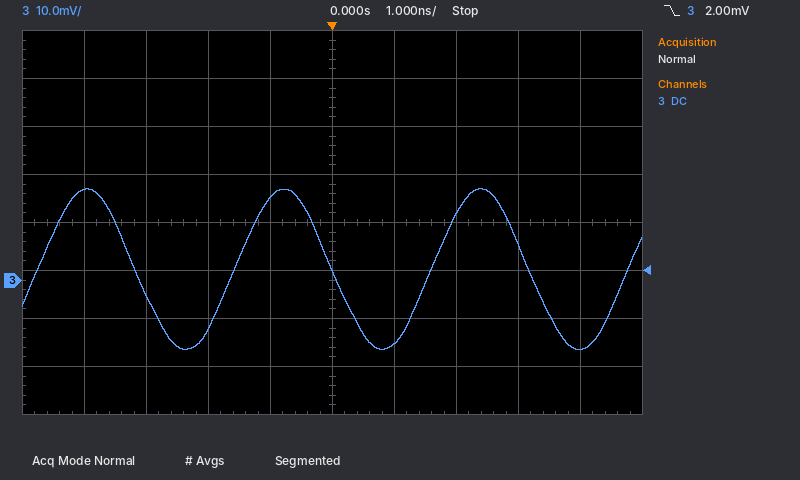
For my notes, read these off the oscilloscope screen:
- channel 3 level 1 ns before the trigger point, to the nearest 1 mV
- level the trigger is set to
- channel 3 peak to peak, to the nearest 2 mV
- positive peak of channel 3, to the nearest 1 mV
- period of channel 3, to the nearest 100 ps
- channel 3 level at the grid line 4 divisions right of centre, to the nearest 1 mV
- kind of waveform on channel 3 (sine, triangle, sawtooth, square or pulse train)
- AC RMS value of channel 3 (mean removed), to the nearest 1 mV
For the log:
17 mV
2.00 mV
34 mV
19 mV
3.2 ns
-14 mV
sine
12 mV
